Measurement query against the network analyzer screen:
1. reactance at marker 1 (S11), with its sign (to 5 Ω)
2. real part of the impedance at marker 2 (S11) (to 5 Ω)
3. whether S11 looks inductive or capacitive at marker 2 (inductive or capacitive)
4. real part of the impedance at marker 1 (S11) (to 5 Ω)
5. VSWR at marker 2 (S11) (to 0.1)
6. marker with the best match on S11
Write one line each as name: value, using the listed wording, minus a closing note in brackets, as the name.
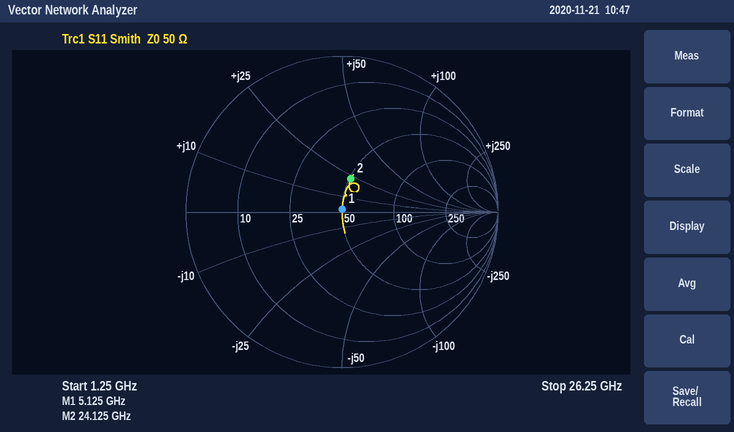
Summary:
reactance at marker 1 (S11), with its sign: 0 Ω
real part of the impedance at marker 2 (S11): 50 Ω
whether S11 looks inductive or capacitive at marker 2: inductive
real part of the impedance at marker 1 (S11): 50 Ω
VSWR at marker 2 (S11): 1.6
marker with the best match on S11: marker 1
